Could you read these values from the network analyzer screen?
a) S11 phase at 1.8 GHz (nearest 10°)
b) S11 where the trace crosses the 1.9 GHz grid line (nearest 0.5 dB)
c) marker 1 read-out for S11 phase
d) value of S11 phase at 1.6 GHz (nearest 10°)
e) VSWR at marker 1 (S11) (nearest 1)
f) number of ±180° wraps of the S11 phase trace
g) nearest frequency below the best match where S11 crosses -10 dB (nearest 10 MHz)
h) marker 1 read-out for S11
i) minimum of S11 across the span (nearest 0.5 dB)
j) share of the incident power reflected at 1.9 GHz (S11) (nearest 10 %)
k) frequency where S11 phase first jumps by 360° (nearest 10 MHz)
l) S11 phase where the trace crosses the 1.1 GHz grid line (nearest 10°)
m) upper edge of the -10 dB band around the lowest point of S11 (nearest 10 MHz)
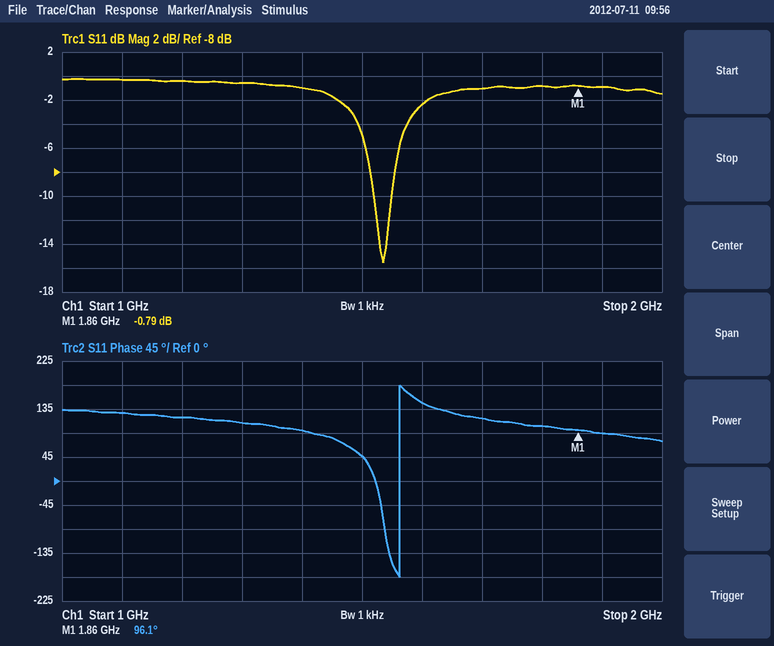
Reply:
100°
-1.0 dB
96.1°
150°
22
1
1.52 GHz
-0.79 dB
-15.5 dB
80 %
1.56 GHz
130°
1.55 GHz
